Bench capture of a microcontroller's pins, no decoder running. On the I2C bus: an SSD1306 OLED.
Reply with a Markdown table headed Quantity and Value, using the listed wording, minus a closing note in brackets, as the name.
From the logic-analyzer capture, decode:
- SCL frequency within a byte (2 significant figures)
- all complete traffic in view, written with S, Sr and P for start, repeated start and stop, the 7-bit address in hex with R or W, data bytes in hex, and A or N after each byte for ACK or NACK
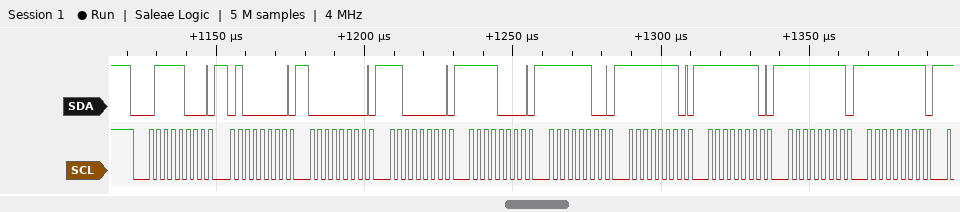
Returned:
| Quantity | Value |
|---|---|
| SCL frequency within a byte | 400 kHz |
| all complete traffic in view, written with S, Sr and P for start, repeated start and stop, the 7-bit address in hex with R or W, data bytes in hex, and A or N after each byte for ACK or NACK | S 3CW A 40 A 00 A C0 A F0 A FC A FE A FE A FF A FF A |
